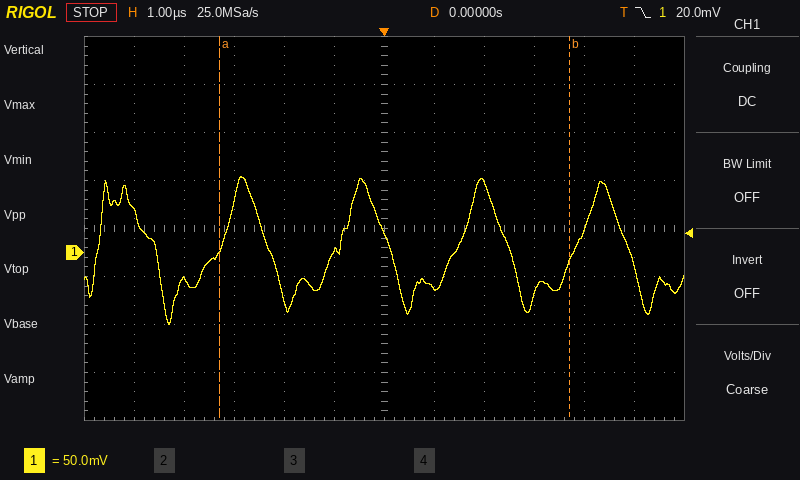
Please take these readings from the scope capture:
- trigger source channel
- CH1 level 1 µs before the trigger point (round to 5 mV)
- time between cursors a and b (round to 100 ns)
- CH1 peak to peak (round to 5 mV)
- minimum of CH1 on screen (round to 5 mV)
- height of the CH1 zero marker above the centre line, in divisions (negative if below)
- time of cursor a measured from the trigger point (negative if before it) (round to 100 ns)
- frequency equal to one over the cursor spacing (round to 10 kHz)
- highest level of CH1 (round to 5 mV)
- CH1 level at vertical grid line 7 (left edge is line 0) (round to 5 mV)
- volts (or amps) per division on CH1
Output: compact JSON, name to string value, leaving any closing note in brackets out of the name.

{"trigger source channel": "CH1", "CH1 level 1 µs before the trigger point": "0 mV", "time between cursors a and b": "7.0 µs", "CH1 peak to peak": "155 mV", "minimum of CH1 on screen": "-75 mV", "height of the CH1 zero marker above the centre line, in divisions": "-0.5 div", "time of cursor a measured from the trigger point (negative if before it)": "-3.3 µs", "frequency equal to one over the cursor spacing": "140 kHz", "highest level of CH1": "80 mV", "CH1 level at vertical grid line 7 (left edge is line 0)": "-35 mV", "volts (or amps) per division on CH1": "50 mV"}
